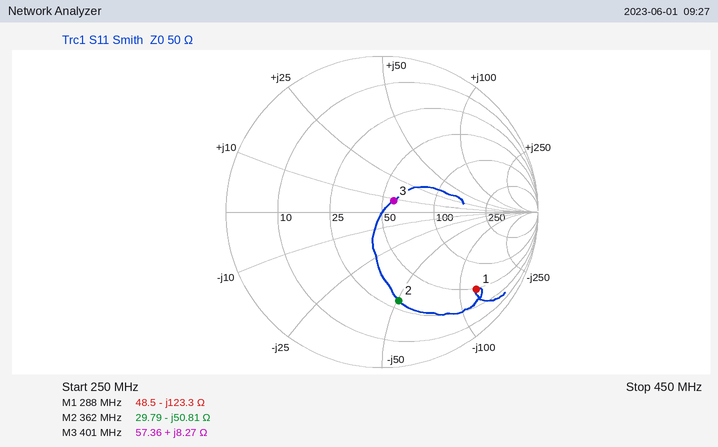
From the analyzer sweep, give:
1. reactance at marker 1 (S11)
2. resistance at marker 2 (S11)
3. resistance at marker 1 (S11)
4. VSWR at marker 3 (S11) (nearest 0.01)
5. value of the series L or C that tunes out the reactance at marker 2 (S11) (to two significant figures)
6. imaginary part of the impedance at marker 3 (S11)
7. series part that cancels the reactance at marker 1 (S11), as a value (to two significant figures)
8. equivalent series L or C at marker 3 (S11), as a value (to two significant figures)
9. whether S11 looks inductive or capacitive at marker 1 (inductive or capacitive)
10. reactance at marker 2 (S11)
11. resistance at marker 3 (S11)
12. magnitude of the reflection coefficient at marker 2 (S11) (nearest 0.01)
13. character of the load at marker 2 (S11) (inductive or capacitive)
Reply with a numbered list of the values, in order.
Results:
1. -123.3 Ω
2. 29.79 Ω
3. 48.5 Ω
4. 1.23
5. 22 nH
6. +8.27 Ω
7. 68 nH
8. 3.3 nH
9. capacitive
10. -50.81 Ω
11. 57.36 Ω
12. 0.58
13. capacitive
